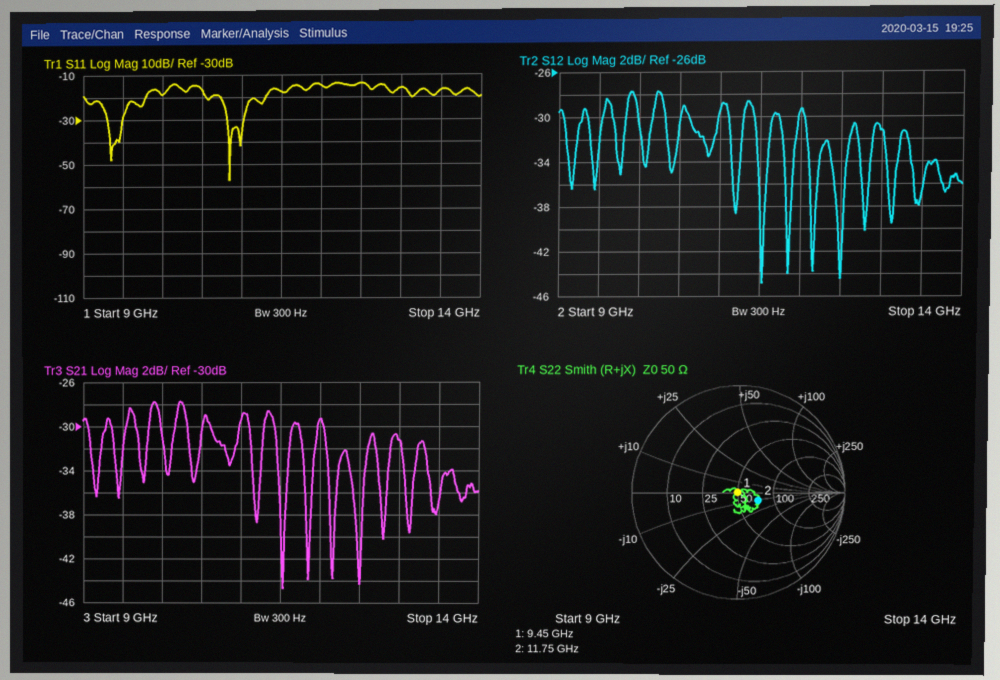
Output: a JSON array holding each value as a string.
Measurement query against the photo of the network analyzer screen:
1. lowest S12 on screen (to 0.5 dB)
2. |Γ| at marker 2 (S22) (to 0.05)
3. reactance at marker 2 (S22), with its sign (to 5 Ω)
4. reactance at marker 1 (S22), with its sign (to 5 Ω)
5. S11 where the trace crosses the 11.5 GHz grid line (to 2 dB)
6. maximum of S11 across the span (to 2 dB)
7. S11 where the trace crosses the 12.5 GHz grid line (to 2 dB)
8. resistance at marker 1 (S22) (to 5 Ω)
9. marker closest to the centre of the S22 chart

["-45.0 dB", "0.20", "-10 Ω", "0 Ω", "-18 dB", "-14 dB", "-14 dB", "50 Ω", "marker 1"]
